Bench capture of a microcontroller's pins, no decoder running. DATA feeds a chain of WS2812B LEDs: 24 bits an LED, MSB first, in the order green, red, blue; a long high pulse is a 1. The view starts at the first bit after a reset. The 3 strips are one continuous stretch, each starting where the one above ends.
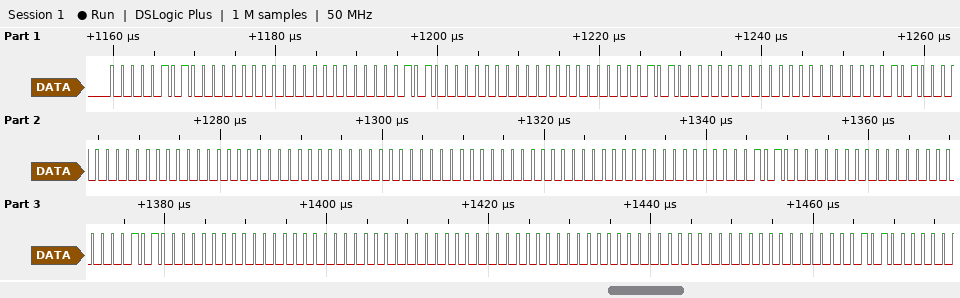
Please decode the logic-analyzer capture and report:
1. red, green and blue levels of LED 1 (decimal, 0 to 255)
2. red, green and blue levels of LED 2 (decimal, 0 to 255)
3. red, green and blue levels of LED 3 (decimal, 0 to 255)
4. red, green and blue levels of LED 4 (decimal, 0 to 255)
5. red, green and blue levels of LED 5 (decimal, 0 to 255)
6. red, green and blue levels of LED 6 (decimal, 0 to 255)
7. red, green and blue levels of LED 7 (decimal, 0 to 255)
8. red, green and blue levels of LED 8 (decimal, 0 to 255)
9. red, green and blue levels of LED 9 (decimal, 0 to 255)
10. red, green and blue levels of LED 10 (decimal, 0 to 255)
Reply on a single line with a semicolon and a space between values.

0, 5, 0; 0, 5, 0; 0, 5, 0; 0, 5, 0; 0, 0, 0; 0, 0, 0; 0, 5, 0; 0, 5, 0; 0, 0, 0; 0, 0, 0
